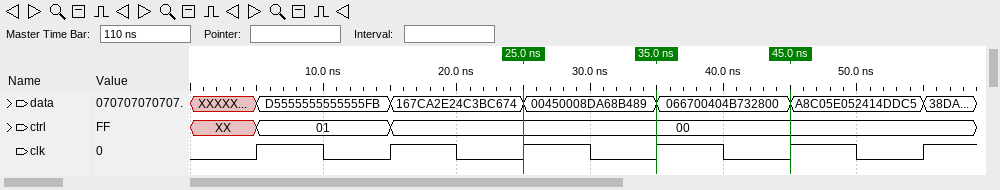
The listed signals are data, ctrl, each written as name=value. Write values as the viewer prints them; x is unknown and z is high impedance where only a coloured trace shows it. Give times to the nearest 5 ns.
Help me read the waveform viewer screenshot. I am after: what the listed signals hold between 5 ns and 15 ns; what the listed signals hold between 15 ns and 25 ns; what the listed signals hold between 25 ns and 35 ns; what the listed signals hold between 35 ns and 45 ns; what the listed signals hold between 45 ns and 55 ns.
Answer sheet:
data=D5555555555555FB, ctrl=01
data=167CA2E24C3BC674, ctrl=00
data=00450008DA68B489, ctrl=00
data=066700404B732800, ctrl=00
data=A8C05E052414DDC5, ctrl=00
